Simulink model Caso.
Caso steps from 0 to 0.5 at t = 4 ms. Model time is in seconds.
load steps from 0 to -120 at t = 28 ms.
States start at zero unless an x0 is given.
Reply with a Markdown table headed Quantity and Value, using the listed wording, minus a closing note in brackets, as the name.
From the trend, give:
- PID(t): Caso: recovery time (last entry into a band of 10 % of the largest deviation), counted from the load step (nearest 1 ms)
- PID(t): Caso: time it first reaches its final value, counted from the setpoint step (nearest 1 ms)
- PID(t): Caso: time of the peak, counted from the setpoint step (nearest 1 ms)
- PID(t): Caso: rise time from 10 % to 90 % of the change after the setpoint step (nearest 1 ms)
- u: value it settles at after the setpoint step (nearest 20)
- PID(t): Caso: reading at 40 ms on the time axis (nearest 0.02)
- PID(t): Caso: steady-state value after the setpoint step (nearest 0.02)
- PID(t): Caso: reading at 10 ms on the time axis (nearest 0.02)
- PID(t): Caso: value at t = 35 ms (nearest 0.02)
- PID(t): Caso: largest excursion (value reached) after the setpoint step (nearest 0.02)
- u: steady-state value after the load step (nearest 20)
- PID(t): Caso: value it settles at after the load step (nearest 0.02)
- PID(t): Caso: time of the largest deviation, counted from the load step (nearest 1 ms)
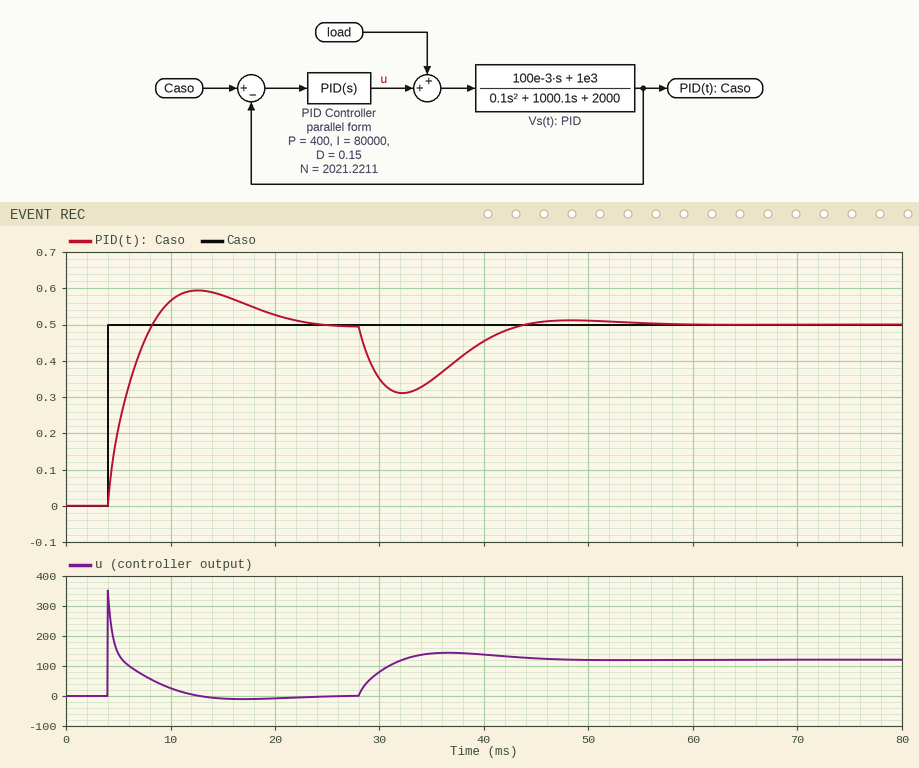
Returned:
| Quantity | Value |
|---|---|
| PID(t): Caso: recovery time (last entry into a band of 10 % of the largest deviation), counted from the load step | 14 ms |
| PID(t): Caso: time it first reaches its final value, counted from the setpoint step | 4 ms |
| PID(t): Caso: time of the peak, counted from the setpoint step | 9 ms |
| PID(t): Caso: rise time from 10 % to 90 % of the change after the setpoint step | 3 ms |
| u: value it settles at after the setpoint step | 0 |
| PID(t): Caso: reading at 40 ms on the time axis | 0.46 |
| PID(t): Caso: steady-state value after the setpoint step | 0.50 |
| PID(t): Caso: reading at 10 ms on the time axis | 0.56 |
| PID(t): Caso: value at t = 35 ms | 0.34 |
| PID(t): Caso: largest excursion (value reached) after the setpoint step | 0.60 |
| u: steady-state value after the load step | 120 |
| PID(t): Caso: value it settles at after the load step | 0.50 |
| PID(t): Caso: time of the largest deviation, counted from the load step | 4 ms |
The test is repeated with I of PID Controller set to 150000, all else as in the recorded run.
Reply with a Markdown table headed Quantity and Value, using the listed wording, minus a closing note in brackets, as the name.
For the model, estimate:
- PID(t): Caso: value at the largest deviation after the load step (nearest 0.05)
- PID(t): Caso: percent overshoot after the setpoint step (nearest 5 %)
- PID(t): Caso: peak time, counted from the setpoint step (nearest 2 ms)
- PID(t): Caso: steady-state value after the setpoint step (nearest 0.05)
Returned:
| Quantity | Value |
|---|---|
| PID(t): Caso: value at the largest deviation after the load step | 0.35 |
| PID(t): Caso: percent overshoot after the setpoint step | 25 % |
| PID(t): Caso: peak time, counted from the setpoint step | 6 ms |
| PID(t): Caso: steady-state value after the setpoint step | 0.50 |
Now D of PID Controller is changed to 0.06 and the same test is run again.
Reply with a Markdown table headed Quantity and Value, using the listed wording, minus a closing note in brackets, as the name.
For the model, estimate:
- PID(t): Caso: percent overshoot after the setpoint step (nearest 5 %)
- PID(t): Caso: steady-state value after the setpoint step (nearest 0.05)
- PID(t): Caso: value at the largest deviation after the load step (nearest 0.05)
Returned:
| Quantity | Value |
|---|---|
| PID(t): Caso: percent overshoot after the setpoint step | 20 % |
| PID(t): Caso: steady-state value after the setpoint step | 0.50 |
| PID(t): Caso: value at the largest deviation after the load step | 0.30 |
